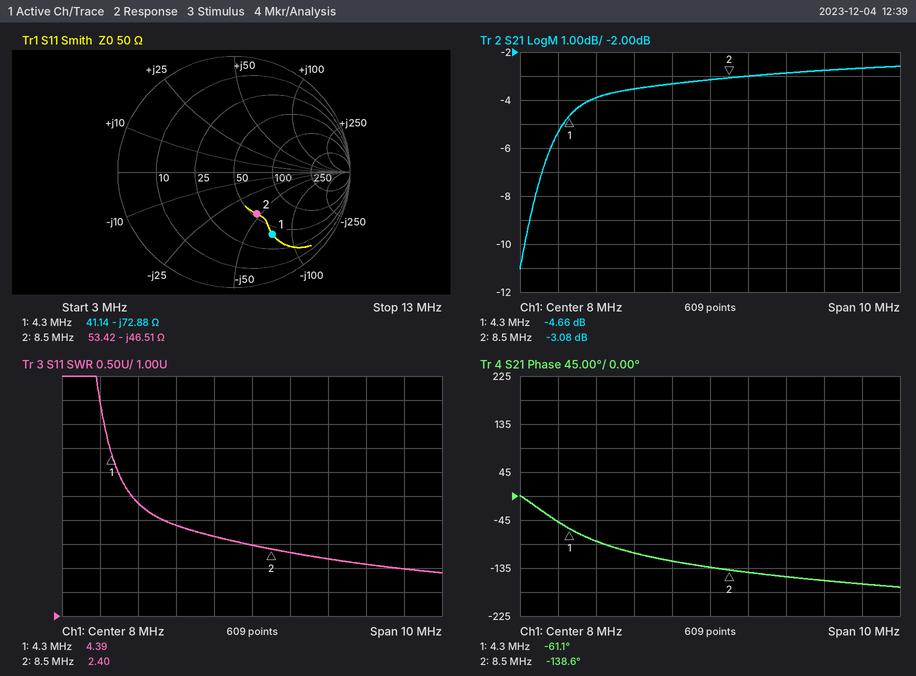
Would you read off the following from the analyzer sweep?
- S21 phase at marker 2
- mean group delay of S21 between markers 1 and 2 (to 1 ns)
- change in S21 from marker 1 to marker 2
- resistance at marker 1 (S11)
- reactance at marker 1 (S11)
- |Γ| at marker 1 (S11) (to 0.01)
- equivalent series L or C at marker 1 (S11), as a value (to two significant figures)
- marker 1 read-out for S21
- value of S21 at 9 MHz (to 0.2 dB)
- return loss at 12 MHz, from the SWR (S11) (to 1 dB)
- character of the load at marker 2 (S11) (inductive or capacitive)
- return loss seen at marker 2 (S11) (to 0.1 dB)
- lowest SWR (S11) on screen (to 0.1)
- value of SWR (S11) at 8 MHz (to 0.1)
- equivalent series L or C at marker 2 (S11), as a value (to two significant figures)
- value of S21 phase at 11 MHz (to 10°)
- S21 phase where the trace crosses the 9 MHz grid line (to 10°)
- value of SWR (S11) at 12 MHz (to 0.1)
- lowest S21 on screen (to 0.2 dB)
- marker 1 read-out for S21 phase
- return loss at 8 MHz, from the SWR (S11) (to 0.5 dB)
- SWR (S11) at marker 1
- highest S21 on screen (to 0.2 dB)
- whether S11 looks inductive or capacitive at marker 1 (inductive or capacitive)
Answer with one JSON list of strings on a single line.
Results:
["-138.6°", "51 ns", "1.58 dB", "41.14 Ω", "-72.88 Ω", "0.63", "510 pF", "-4.66 dB", "-3.0 dB", "10 dB", "capacitive", "7.7 dB", "1.9", "2.5", "400 pF", "-160°", "-140°", "2.0", "-11.0 dB", "-61.1°", "7.5 dB", "4.39", "-2.6 dB", "capacitive"]
